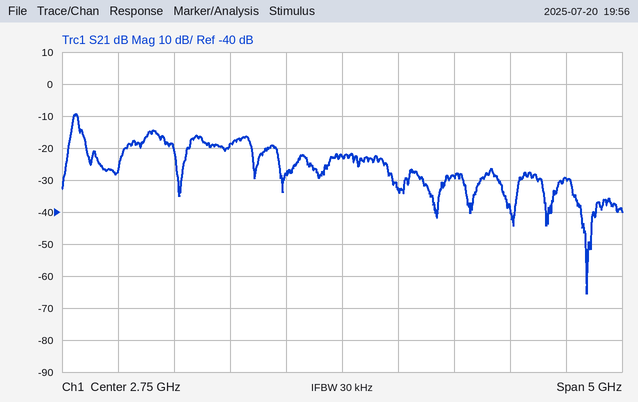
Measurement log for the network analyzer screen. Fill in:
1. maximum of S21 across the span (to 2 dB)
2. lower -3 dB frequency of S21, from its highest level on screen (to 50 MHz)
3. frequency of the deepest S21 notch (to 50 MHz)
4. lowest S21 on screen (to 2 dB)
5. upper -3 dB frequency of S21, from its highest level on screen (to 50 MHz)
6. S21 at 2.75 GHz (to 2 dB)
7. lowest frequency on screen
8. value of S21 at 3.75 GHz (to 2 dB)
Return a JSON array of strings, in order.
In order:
["-10 dB", "350 MHz", "4.95 GHz", "-66 dB", "400 MHz", "-22 dB", "250 MHz", "-28 dB"]
